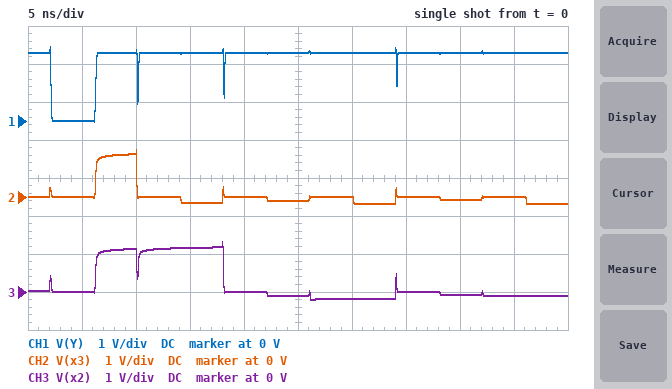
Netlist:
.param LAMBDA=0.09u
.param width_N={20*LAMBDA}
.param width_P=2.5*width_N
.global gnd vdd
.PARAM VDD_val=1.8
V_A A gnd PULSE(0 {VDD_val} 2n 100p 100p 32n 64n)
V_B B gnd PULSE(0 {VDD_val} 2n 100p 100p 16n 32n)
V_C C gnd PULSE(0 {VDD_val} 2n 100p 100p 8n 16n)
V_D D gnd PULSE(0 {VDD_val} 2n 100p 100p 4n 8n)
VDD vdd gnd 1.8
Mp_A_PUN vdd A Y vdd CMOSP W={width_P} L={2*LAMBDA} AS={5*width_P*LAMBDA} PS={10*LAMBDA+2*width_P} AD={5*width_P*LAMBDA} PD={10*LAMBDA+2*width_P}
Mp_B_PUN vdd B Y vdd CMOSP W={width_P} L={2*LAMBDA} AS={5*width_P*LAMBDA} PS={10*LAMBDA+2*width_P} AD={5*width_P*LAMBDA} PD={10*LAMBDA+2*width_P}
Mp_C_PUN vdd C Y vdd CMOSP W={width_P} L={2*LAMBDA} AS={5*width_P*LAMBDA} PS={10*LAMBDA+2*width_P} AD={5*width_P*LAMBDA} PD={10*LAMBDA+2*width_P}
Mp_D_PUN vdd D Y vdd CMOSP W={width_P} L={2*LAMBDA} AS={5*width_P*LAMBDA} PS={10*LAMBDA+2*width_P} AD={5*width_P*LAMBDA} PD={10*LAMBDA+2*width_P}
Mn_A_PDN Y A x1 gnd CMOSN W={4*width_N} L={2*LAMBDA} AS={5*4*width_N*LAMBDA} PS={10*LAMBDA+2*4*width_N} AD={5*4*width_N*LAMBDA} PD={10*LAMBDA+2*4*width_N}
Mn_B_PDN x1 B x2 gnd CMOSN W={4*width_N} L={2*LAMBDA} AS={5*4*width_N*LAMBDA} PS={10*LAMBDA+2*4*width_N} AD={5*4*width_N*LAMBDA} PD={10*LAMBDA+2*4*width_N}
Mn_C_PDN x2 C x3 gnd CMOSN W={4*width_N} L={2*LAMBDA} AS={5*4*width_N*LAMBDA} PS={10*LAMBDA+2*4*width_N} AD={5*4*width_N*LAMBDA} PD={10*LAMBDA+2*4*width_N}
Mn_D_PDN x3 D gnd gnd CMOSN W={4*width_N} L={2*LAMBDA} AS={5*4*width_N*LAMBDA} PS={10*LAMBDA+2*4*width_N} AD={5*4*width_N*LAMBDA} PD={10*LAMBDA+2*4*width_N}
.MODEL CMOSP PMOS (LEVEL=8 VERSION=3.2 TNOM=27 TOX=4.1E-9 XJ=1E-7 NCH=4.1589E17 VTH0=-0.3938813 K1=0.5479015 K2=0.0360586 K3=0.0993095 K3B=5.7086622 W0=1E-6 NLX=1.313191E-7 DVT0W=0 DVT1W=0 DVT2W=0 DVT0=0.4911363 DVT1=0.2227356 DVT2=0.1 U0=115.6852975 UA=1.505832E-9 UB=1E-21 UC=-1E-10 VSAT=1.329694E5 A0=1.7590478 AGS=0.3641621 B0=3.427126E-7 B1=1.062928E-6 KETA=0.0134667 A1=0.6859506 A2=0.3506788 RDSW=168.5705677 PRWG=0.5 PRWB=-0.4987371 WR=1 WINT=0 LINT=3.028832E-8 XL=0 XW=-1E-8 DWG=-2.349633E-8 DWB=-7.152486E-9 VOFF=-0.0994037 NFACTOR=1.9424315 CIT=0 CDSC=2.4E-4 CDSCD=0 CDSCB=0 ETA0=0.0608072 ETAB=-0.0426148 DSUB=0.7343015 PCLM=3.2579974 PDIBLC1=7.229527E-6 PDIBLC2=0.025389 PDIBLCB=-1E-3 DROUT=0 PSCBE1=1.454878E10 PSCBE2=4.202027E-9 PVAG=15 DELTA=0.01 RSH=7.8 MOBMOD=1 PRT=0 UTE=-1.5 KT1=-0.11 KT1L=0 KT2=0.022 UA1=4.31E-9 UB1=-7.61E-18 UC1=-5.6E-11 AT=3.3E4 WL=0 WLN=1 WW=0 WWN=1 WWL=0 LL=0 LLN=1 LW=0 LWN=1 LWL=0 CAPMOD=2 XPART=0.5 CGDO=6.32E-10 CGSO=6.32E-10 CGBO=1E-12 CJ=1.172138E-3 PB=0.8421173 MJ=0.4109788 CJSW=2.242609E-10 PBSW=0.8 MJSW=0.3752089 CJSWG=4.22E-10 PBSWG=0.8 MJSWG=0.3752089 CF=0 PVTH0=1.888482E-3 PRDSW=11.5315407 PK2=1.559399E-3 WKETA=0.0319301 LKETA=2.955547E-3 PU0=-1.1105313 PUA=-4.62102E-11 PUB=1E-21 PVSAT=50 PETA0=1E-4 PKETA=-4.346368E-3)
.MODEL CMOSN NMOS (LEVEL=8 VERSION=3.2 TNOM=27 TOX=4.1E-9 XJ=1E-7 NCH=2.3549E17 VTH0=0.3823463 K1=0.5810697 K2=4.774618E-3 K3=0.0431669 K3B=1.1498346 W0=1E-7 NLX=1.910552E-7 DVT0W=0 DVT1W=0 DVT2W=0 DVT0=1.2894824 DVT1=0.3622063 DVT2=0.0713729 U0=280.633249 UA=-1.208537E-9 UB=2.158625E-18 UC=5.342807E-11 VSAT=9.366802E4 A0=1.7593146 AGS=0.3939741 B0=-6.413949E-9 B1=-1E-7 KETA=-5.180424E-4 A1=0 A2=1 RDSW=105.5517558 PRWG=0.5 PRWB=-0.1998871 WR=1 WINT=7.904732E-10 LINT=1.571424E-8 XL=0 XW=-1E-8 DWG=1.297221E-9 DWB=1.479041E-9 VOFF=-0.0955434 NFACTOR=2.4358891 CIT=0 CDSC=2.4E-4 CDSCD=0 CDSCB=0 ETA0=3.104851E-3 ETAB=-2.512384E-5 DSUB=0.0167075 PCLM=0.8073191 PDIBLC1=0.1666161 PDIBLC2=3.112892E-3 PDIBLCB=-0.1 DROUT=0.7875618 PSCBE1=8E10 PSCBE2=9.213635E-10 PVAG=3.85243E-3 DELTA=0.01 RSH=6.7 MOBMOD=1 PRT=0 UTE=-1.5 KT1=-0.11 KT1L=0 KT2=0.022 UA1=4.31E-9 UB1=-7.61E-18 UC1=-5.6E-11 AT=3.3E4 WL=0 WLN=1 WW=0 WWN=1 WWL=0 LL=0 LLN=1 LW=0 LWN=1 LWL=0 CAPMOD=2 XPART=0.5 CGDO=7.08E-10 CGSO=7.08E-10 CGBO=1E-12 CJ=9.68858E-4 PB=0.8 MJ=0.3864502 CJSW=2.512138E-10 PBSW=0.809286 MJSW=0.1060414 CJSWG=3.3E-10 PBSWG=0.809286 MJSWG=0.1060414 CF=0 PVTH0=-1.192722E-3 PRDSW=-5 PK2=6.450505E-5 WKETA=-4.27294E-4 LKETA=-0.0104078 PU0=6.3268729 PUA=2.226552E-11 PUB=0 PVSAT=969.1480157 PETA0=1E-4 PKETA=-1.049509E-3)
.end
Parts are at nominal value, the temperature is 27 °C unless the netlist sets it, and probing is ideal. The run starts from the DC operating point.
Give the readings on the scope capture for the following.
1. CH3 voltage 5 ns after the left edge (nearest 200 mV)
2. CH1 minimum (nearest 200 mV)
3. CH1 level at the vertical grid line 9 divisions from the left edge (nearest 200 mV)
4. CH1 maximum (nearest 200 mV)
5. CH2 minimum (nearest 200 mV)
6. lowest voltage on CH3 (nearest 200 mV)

0 V
0 V
1.8 V
2.0 V
-200 mV
-200 mV
